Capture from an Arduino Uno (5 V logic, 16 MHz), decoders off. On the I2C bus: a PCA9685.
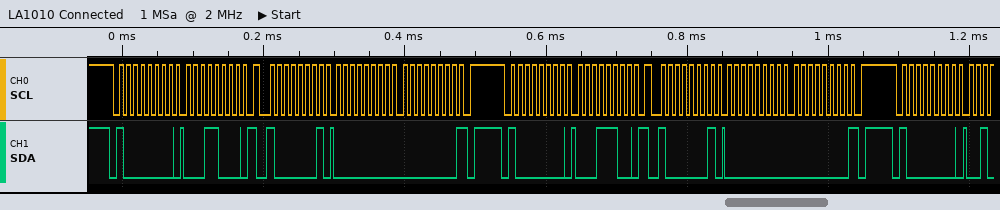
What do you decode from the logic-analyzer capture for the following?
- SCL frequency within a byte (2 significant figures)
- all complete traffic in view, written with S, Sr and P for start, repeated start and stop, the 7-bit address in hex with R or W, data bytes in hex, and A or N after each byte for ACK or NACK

100 kHz
S 40W A 18 A Sr 40R A 00 A 00 N P S 40W A 1C A Sr 40R A 00 A 00 N P S 40W A
